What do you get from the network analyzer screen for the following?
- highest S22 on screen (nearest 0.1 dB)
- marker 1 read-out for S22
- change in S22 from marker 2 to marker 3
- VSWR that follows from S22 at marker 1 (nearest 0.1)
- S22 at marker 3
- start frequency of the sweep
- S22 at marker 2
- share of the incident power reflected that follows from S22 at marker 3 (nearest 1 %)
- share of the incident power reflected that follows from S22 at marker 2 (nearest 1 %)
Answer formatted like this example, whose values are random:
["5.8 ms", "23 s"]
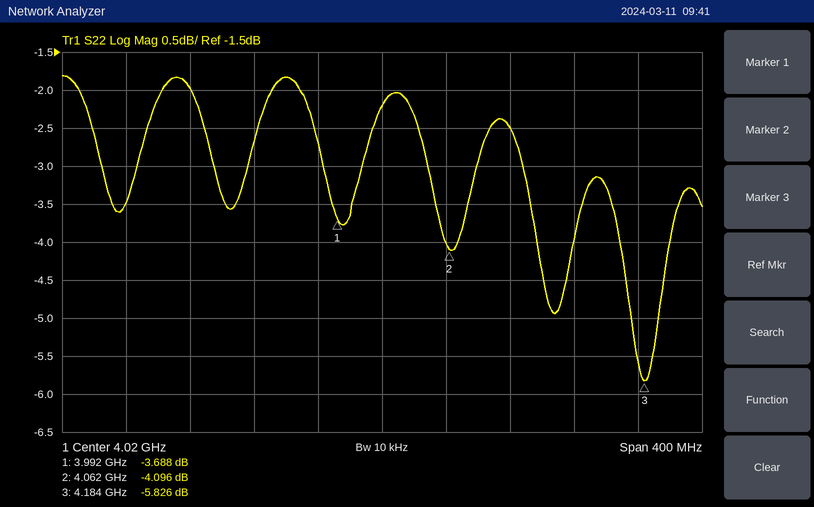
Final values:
["-1.8 dB", "-3.688 dB", "-1.730 dB", "4.8", "-5.826 dB", "3.82 GHz", "-4.096 dB", "26 %", "39 %"]
